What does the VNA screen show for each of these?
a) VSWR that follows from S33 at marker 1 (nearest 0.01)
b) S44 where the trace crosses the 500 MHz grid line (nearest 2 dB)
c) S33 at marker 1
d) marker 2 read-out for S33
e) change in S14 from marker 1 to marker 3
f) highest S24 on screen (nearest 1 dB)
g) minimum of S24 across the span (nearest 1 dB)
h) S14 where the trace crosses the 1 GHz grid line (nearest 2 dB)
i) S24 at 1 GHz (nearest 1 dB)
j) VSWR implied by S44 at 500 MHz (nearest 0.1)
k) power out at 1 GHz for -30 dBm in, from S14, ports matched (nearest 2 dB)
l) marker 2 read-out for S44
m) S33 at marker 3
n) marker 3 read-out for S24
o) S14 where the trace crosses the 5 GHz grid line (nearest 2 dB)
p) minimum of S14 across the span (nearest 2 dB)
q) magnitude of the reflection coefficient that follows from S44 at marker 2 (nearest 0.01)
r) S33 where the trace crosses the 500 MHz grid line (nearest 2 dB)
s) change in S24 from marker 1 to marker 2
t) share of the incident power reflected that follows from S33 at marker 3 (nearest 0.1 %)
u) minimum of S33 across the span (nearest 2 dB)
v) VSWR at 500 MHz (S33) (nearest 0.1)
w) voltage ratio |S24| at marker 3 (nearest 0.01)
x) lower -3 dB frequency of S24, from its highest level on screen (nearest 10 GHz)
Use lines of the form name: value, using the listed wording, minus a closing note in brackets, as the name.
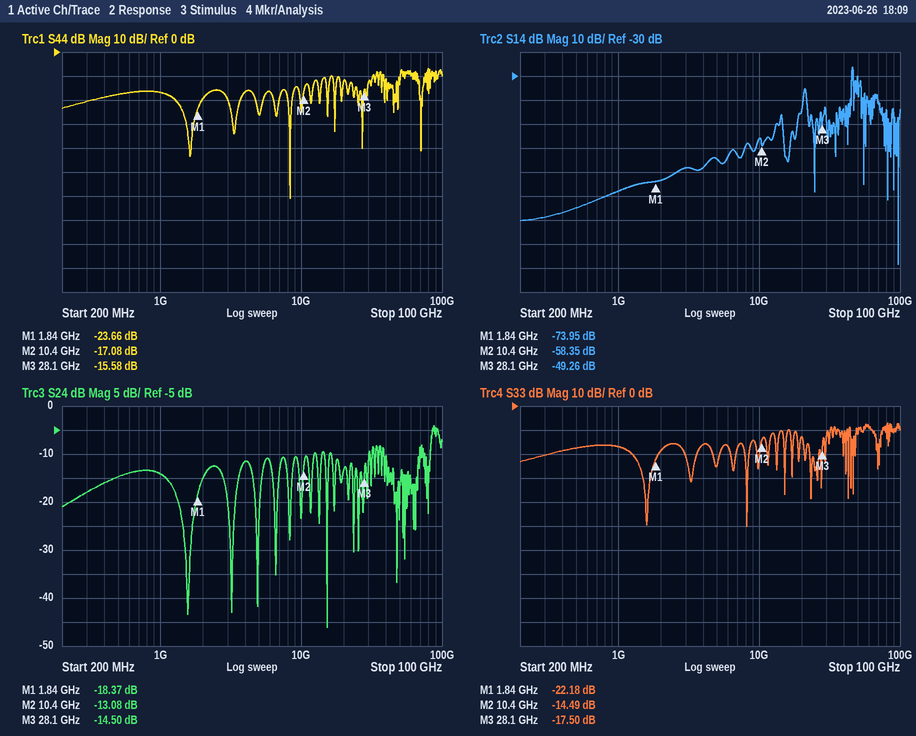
VSWR that follows from S33 at marker 1: 1.17
S44 where the trace crosses the 500 MHz grid line: -18 dB
S33 at marker 1: -22.18 dB
marker 2 read-out for S33: -14.49 dB
change in S14 from marker 1 to marker 3: 24.69 dB
highest S24 on screen: -4 dB
minimum of S24 across the span: -46 dB
S14 where the trace crosses the 1 GHz grid line: -78 dB
S24 at 1 GHz: -14 dB
VSWR implied by S44 at 500 MHz: 1.3
power out at 1 GHz for -30 dBm in, from S14, ports matched: -108 dBm
marker 2 read-out for S44: -17.08 dB
S33 at marker 3: -17.50 dB
marker 3 read-out for S24: -14.50 dB
S14 where the trace crosses the 5 GHz grid line: -64 dB
minimum of S14 across the span: -108 dB
magnitude of the reflection coefficient that follows from S44 at marker 2: 0.14
S33 where the trace crosses the 500 MHz grid line: -18 dB
change in S24 from marker 1 to marker 2: 5.29 dB
share of the incident power reflected that follows from S33 at marker 3: 1.8 %
minimum of S33 across the span: -50 dB
VSWR at 500 MHz (S33): 1.3
voltage ratio |S24| at marker 3: 0.19
lower -3 dB frequency of S24, from its highest level on screen: 80 GHz
